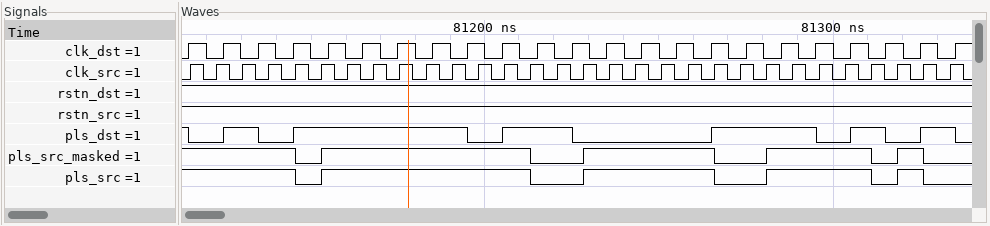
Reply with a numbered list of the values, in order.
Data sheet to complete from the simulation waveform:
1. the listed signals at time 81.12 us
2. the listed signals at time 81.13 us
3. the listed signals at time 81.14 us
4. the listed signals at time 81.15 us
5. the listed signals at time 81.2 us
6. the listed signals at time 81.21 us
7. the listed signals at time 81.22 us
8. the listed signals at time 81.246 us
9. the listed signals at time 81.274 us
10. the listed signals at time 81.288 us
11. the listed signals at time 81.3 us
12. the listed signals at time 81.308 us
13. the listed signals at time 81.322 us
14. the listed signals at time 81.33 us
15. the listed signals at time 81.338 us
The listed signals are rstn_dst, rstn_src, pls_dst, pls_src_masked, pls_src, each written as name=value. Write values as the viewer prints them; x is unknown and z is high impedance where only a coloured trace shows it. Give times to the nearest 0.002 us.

1. rstn_dst=1, rstn_src=1, pls_dst=0, pls_src_masked=1, pls_src=1
2. rstn_dst=1, rstn_src=1, pls_dst=1, pls_src_masked=1, pls_src=1
3. rstn_dst=1, rstn_src=1, pls_dst=0, pls_src_masked=1, pls_src=1
4. rstn_dst=1, rstn_src=1, pls_dst=1, pls_src_masked=0, pls_src=0
5. rstn_dst=1, rstn_src=1, pls_dst=0, pls_src_masked=1, pls_src=1
6. rstn_dst=1, rstn_src=1, pls_dst=1, pls_src_masked=1, pls_src=1
7. rstn_dst=1, rstn_src=1, pls_dst=1, pls_src_masked=0, pls_src=0
8. rstn_dst=1, rstn_src=1, pls_dst=0, pls_src_masked=1, pls_src=1
9. rstn_dst=1, rstn_src=1, pls_dst=1, pls_src_masked=0, pls_src=0
10. rstn_dst=1, rstn_src=1, pls_dst=1, pls_src_masked=1, pls_src=1
11. rstn_dst=1, rstn_src=1, pls_dst=0, pls_src_masked=1, pls_src=1
12. rstn_dst=1, rstn_src=1, pls_dst=1, pls_src_masked=1, pls_src=1
13. rstn_dst=1, rstn_src=1, pls_dst=0, pls_src_masked=1, pls_src=1
14. rstn_dst=1, rstn_src=1, pls_dst=1, pls_src_masked=0, pls_src=0
15. rstn_dst=1, rstn_src=1, pls_dst=0, pls_src_masked=0, pls_src=0
